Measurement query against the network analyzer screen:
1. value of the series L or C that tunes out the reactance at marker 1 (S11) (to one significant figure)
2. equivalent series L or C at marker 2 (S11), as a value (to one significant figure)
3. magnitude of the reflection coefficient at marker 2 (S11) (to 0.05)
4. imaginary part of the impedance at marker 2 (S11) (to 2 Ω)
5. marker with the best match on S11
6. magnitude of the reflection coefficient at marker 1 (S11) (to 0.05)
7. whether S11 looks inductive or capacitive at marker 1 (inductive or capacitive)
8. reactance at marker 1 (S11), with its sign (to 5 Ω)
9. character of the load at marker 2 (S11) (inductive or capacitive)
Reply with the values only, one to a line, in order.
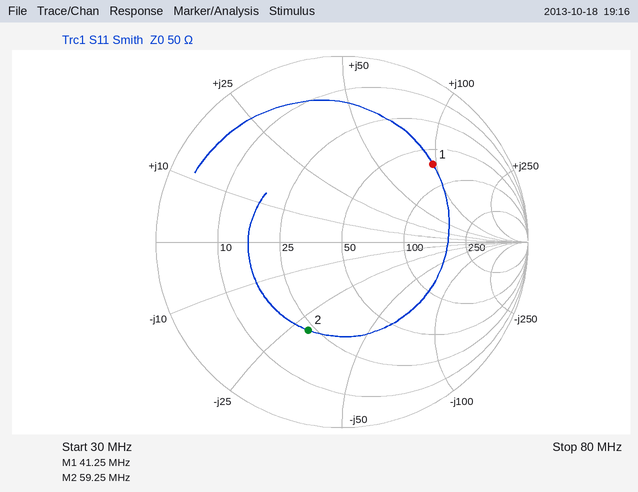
40 pF
90 pF
0.50
-30 Ω
marker 2
0.65
inductive
+95 Ω
capacitive
